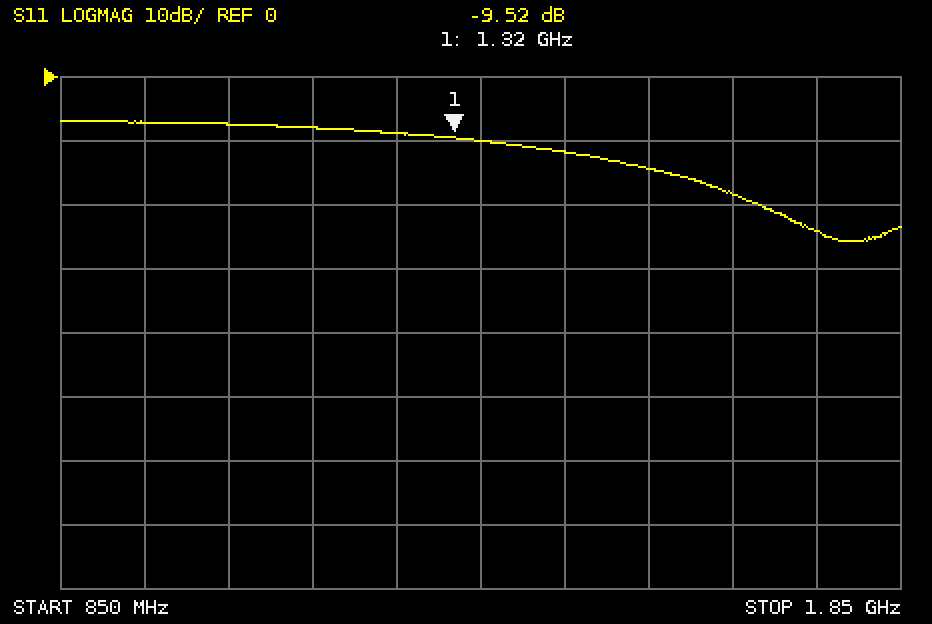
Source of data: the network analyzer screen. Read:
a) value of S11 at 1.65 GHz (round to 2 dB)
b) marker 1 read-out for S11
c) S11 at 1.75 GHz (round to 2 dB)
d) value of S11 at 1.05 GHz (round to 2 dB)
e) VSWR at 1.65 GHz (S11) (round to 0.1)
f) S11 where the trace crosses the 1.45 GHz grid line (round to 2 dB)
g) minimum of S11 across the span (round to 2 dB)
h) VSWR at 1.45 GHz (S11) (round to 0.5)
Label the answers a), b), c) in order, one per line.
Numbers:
a) -18 dB
b) -9.52 dB
c) -24 dB
d) -8 dB
e) 1.3
f) -12 dB
g) -26 dB
h) 1.5
